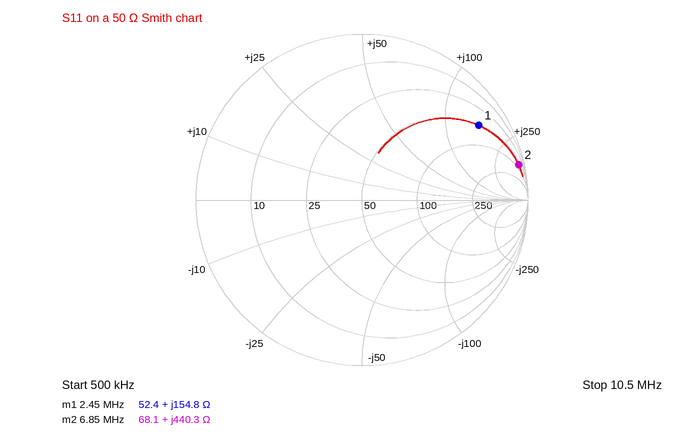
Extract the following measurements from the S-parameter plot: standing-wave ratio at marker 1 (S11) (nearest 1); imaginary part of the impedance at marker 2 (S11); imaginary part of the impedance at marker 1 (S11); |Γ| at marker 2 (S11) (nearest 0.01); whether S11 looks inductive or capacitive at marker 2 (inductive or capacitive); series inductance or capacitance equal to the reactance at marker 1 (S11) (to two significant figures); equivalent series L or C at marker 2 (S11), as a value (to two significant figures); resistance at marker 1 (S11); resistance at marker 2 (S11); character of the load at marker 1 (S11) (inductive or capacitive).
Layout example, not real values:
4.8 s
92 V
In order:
11
+440.3 Ω
+154.8 Ω
0.97
inductive
10 µH
10 µH
52.4 Ω
68.1 Ω
inductive
